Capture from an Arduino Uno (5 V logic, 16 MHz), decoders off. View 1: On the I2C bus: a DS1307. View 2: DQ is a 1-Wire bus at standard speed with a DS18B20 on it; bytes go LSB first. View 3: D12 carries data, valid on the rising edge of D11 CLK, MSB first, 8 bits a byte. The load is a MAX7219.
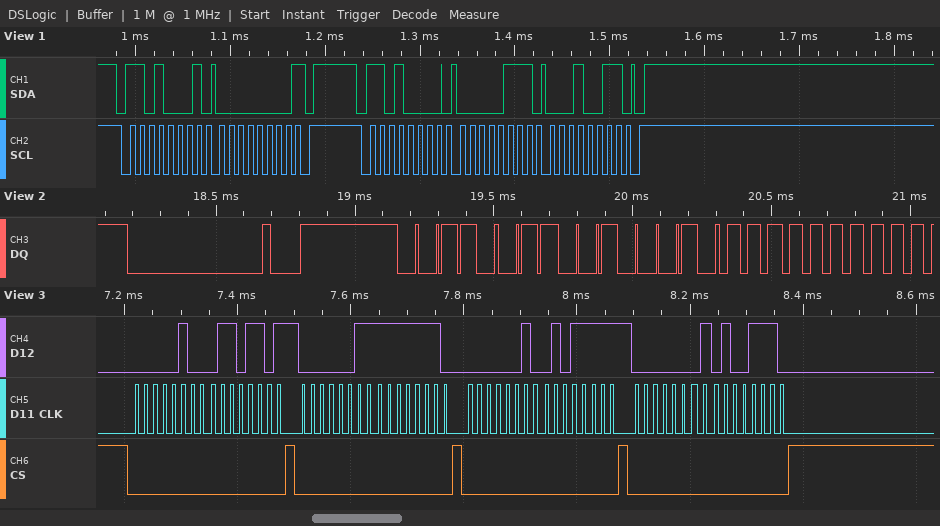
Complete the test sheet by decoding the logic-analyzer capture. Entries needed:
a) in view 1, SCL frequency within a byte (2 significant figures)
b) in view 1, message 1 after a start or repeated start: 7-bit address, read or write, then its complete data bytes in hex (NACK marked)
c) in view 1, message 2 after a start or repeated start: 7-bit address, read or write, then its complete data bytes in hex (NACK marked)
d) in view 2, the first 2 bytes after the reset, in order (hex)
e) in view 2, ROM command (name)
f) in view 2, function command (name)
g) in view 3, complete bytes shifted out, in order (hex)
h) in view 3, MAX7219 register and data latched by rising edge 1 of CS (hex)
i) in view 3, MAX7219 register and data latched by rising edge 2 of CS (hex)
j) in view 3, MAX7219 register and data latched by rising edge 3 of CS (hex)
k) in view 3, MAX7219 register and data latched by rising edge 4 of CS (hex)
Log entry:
100 kHz
0x68 read: 00 NACK
0x68 write: 07 13
CC 44
Skip ROM
Convert T
04 6D 03 FE 02 5F 01 4E
register 0x4, data 0x6D
register 0x3, data 0xFE
register 0x2, data 0x5F
register 0x1, data 0x4E
